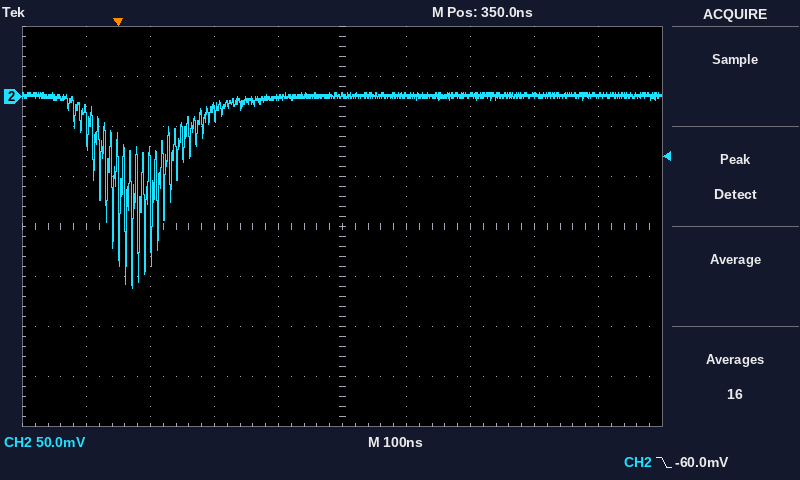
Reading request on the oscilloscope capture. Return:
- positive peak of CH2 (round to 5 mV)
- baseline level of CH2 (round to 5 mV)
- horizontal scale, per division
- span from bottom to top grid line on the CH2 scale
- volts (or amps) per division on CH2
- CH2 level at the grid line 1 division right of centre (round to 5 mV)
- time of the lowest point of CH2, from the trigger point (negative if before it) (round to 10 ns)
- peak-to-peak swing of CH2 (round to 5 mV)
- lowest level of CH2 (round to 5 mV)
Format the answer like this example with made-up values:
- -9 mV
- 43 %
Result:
- 5 mV
- 0 mV
- 100 ns
- 400 mV
- 50 mV
- 0 mV
- +20 ns
- 195 mV
- -190 mV
